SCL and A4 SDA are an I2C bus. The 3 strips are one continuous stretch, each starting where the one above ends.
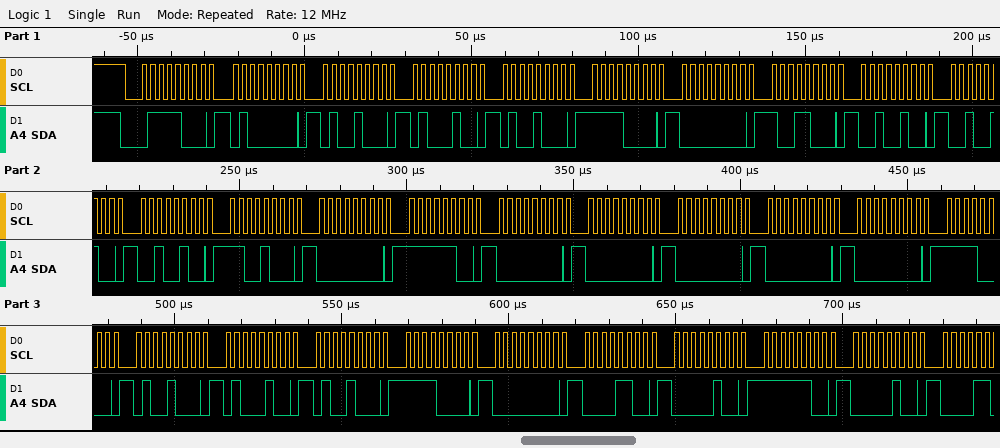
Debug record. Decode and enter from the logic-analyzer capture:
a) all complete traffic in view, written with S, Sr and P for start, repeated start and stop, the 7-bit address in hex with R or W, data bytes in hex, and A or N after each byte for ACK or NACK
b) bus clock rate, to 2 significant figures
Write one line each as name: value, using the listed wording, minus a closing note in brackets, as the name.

all complete traffic in view, written with S, Sr and P for start, repeated start and stop, the 7-bit address in hex with R or W, data bytes in hex, and A or N after each byte for ACK or NACK: S 3CW A 40 A 48 A 44 A 48 A F0 A 00 A 98 A 24 A 24 A 24 A C8 A 00 A FC A 00 A 00 A 00 A 00 A 00 A F0 A 48 A 44 A 48 A F0 A 00 A 0C A 04 A FC A 04 A
bus clock rate, to 2 significant figures: 400 kHz
